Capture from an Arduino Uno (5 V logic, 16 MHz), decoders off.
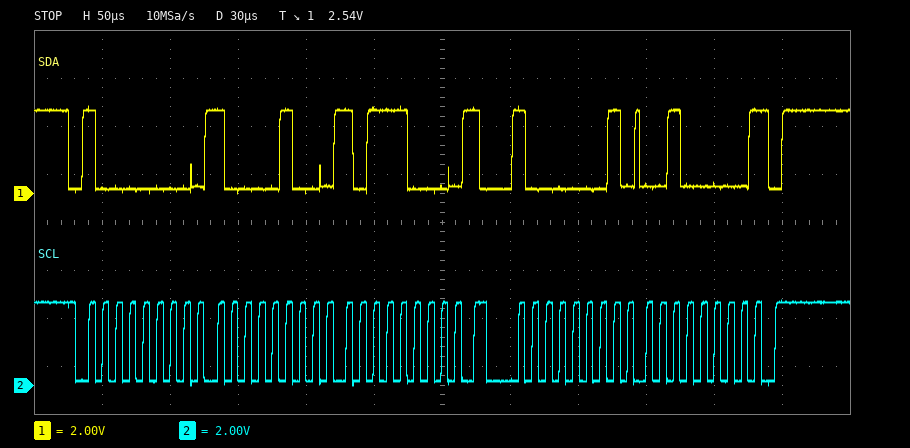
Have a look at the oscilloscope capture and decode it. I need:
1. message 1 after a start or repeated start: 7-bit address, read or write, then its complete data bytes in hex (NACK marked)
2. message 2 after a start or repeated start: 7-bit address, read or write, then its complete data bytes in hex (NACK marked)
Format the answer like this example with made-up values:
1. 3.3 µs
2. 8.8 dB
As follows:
1. 0x40 write: 84 B8
2. 0x40 read: 20 NACK
